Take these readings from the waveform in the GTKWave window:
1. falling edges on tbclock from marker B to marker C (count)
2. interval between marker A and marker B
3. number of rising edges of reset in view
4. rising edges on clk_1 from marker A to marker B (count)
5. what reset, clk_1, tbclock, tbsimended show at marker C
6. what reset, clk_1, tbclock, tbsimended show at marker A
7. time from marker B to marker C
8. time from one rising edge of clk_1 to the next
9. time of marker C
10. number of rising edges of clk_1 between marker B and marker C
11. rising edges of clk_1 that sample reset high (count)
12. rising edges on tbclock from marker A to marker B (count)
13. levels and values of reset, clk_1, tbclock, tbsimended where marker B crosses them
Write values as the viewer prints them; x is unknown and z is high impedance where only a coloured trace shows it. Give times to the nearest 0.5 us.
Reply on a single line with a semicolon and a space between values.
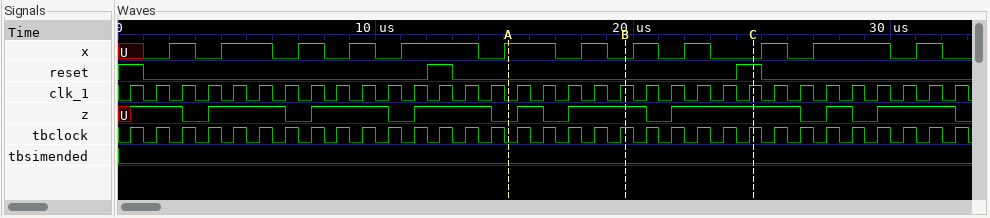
5; 4.5 us; 2; 5; reset=1, clk_1=1, tbclock=1, tbsimended=0; reset=0, clk_1=0, tbclock=0, tbsimended=0; 5 us; 1 us; 24.5 us; 5; 3; 5; reset=0, clk_1=1, tbclock=1, tbsimended=0
